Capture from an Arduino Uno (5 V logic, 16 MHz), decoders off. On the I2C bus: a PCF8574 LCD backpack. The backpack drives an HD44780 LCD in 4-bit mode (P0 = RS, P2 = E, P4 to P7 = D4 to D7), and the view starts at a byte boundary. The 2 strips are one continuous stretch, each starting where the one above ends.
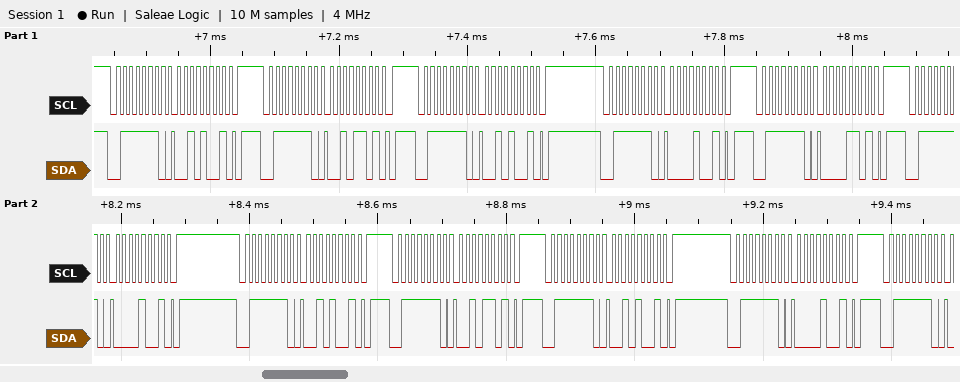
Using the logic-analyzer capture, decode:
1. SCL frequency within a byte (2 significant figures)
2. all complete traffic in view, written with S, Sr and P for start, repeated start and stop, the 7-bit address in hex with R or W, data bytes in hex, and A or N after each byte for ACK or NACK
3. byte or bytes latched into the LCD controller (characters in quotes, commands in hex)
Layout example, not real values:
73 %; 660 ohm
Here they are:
100 kHz; S 3FW A 29 A P S 3FW A 2D A P S 3FW A 29 A P S 3FW A 09 A P S 3FW A 0D A P S 3FW A 09 A P S 3FW A 29 A P S 3FW A 2D A P S 3FW A 29 A P S 3FW A 09 A P S 3FW A; ' '
